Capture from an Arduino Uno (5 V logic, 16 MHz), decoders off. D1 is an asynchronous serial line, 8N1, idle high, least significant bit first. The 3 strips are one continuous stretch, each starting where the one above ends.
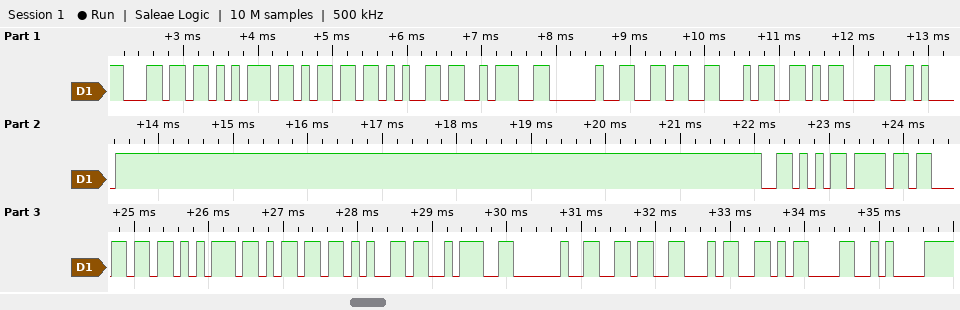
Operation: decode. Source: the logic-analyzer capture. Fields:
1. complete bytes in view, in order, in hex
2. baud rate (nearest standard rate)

6C 75 6D 65 3A 20 36 34 0D 0A 56 6F 6C 75 6D 65 3A 20 36 34 0D 0A
9600 baud
